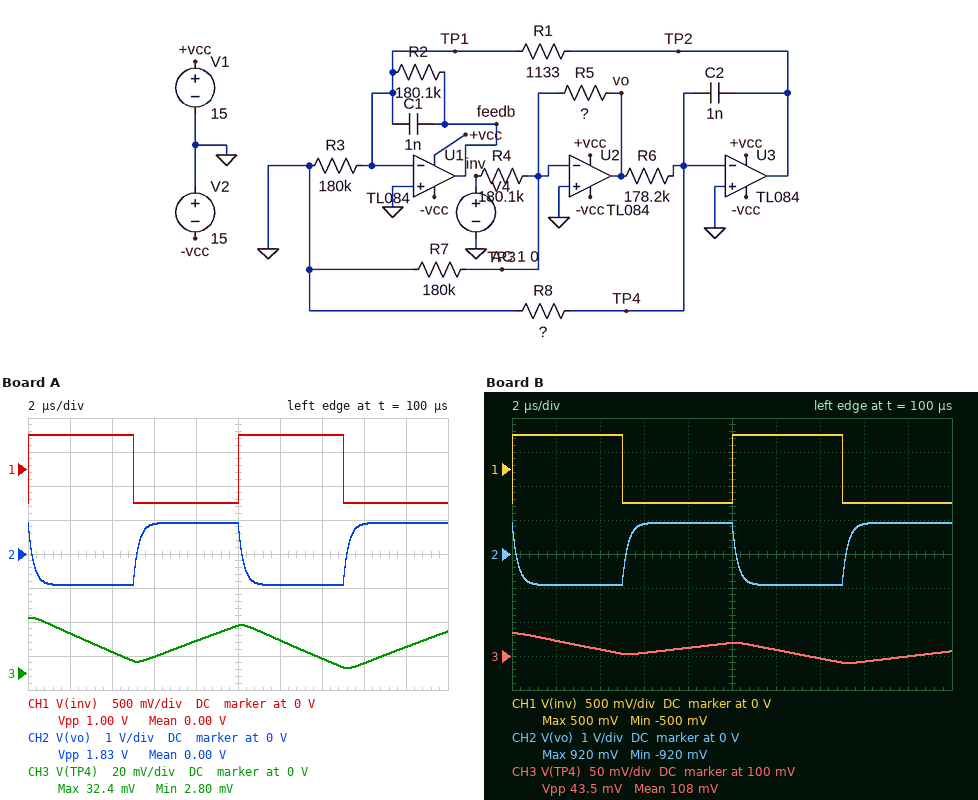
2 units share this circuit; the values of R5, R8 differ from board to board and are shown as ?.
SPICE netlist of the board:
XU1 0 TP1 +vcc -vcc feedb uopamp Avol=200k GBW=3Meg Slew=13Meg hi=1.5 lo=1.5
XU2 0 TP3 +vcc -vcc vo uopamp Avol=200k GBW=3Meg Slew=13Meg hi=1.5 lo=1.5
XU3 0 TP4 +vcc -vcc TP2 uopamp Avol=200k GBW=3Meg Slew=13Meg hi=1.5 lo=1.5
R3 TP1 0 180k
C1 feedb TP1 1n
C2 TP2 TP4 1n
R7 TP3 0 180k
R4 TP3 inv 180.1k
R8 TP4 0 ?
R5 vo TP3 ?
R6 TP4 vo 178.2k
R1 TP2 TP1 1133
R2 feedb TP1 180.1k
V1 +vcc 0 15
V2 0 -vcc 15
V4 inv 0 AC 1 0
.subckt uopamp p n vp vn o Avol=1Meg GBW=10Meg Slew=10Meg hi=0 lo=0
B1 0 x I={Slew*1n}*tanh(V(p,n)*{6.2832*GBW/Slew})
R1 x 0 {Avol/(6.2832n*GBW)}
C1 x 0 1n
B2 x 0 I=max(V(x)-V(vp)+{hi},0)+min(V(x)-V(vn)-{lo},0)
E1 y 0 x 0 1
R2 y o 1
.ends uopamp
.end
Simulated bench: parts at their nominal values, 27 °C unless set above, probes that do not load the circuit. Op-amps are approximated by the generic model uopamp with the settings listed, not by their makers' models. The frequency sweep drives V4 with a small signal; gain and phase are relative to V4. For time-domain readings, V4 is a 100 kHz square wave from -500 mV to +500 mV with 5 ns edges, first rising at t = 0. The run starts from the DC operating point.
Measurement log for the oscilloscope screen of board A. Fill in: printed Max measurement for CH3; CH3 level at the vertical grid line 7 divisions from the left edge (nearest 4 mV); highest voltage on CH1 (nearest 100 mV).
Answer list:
32.4 mV
8 mV
500 mV
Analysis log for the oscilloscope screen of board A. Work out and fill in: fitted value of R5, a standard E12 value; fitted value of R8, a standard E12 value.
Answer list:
330 kΩ
56 kΩ
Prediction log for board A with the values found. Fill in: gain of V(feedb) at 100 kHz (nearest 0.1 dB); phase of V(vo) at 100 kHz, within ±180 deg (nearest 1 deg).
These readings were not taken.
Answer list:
-33.3 dB
171 deg
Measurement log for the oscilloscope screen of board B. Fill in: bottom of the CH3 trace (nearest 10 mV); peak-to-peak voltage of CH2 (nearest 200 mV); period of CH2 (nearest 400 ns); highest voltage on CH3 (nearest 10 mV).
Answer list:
90 mV
1.8 V
10.0 µs
130 mV
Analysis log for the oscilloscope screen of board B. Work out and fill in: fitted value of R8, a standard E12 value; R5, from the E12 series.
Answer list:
150 kΩ
330 kΩ
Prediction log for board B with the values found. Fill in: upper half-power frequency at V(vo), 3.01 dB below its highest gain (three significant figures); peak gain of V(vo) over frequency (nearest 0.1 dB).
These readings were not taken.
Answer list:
643 kHz
5.3 dB
